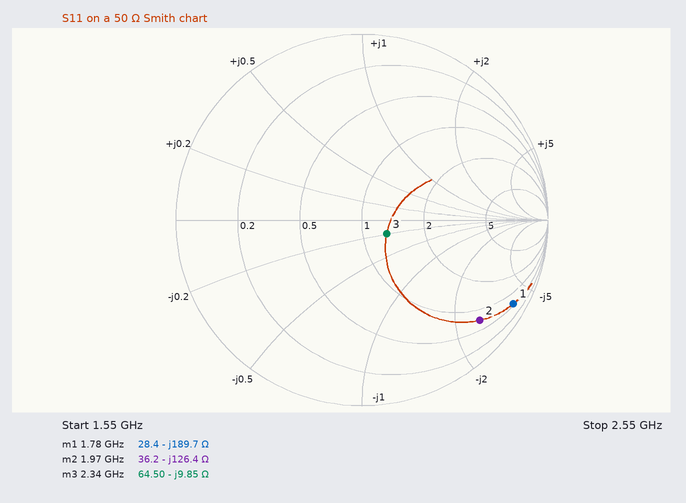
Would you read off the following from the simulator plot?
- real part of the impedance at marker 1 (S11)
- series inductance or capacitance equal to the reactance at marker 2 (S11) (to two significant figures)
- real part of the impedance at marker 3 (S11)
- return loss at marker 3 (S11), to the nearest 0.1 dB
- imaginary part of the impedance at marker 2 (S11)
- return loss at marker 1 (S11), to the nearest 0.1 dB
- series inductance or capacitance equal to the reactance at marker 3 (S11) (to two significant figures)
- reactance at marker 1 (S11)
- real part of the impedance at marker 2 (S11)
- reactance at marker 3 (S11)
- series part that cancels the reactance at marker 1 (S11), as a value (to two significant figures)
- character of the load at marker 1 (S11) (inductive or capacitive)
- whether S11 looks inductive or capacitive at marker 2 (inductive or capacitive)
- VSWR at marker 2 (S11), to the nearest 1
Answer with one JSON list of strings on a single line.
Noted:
["28.4 Ω", "640 fF", "64.50 Ω", "16.3 dB", "-126.4 Ω", "0.6 dB", "6.9 pF", "-189.7 Ω", "36.2 Ω", "-9.85 Ω", "17 nH", "capacitive", "capacitive", "11"]
